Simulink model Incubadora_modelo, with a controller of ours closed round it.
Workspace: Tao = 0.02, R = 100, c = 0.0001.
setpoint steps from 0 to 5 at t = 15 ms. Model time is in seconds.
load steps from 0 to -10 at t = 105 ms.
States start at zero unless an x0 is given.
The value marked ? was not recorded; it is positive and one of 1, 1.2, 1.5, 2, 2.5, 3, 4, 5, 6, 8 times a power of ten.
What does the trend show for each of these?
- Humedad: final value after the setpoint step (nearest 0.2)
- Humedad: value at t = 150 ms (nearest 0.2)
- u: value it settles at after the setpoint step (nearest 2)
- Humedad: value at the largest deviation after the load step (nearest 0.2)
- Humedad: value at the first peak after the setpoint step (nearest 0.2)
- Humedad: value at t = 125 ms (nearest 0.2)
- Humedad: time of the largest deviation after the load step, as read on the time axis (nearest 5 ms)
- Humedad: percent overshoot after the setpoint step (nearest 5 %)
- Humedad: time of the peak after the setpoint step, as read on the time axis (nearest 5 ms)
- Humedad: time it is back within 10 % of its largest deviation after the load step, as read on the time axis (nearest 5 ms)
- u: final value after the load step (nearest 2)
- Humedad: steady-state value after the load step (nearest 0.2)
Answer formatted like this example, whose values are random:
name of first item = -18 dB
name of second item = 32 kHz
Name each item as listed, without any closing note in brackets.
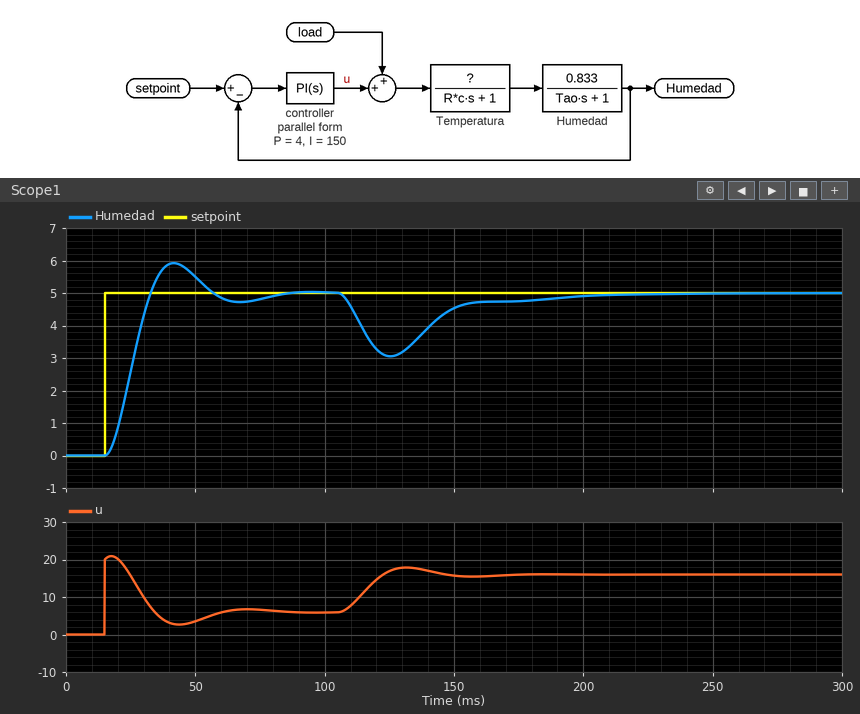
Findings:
Humedad: final value after the setpoint step = 5.0
Humedad: value at t = 150 ms = 4.6
u: value it settles at after the setpoint step = 6
Humedad: value at the largest deviation after the load step = 3.0
Humedad: value at the first peak after the setpoint step = 6.0
Humedad: value at t = 125 ms = 3.0
Humedad: time of the largest deviation after the load step, as read on the time axis = 125 ms
Humedad: percent overshoot after the setpoint step = 20 %
Humedad: time of the peak after the setpoint step, as read on the time axis = 40 ms
Humedad: time it is back within 10 % of its largest deviation after the load step, as read on the time axis = 185 ms
u: final value after the load step = 16
Humedad: steady-state value after the load step = 5.0
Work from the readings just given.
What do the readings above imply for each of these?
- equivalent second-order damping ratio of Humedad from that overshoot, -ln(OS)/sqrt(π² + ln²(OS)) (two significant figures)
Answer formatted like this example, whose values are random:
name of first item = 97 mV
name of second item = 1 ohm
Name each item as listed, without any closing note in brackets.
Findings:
equivalent second-order damping ratio of Humedad from that overshoot, -ln(OS)/sqrt(π² + ln²(OS)) = 0.46
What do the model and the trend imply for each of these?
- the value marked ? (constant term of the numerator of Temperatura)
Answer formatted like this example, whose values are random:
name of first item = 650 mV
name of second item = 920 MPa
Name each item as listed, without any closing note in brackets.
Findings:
the value marked ? = 1
